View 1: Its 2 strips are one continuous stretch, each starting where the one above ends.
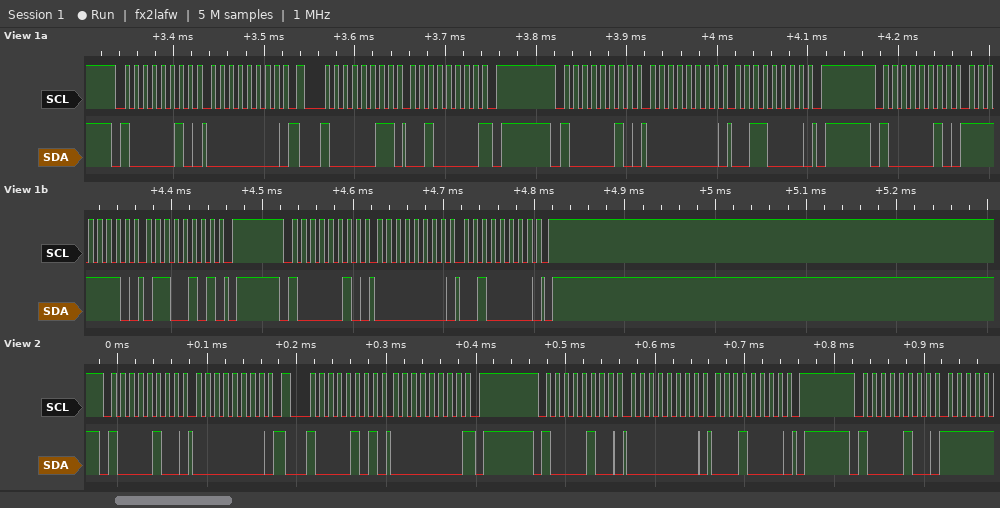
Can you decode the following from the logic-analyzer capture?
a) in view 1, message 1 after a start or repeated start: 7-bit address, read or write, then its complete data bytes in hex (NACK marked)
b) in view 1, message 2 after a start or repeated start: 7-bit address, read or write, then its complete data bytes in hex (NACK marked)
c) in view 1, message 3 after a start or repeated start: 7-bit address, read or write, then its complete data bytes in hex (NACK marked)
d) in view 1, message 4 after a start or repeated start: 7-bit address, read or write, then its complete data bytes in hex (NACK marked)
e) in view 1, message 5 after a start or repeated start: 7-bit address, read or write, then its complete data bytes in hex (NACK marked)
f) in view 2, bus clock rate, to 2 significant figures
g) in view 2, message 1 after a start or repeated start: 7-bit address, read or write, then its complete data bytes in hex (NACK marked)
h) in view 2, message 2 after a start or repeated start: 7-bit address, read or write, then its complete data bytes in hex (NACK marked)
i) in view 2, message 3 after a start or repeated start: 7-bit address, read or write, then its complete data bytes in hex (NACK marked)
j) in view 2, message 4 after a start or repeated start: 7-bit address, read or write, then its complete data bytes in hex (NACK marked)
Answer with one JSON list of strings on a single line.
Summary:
["0x41 write: 00", "0x41 read: 20 NACK", "0x41 write: 00 30", "0x41 write: FE 65", "0x41 write: 00 20", "100 kHz", "0x42 write: 00", "0x42 read: 00 NACK", "0x42 write: 00 10", "0x42 write"]
